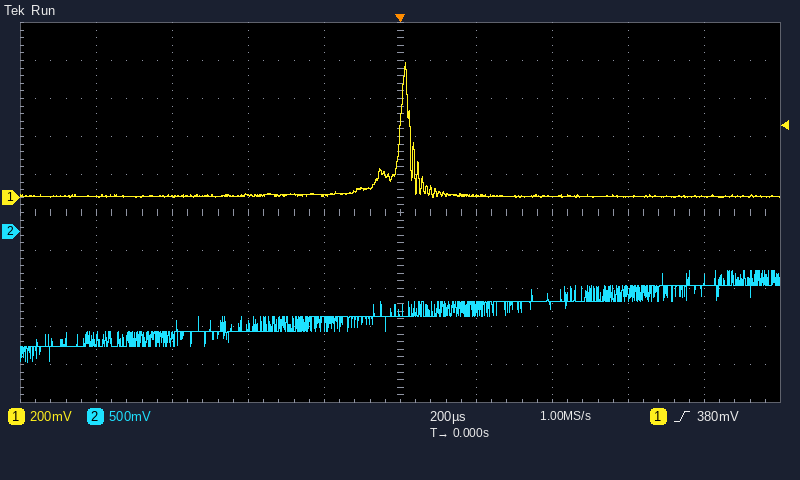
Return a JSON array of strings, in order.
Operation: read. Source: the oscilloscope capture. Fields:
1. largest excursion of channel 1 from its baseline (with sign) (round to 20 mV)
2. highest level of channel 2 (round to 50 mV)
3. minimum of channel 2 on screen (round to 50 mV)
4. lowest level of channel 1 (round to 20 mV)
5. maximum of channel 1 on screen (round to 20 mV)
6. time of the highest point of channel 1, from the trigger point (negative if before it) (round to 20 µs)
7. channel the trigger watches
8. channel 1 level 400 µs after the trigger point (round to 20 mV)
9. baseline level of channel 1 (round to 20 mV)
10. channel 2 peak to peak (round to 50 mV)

["+700 mV", "-500 mV", "-1.70 V", "0 mV", "700 mV", "+20 µs", "channel 1", "0 mV", "0 mV", "1.20 V"]
